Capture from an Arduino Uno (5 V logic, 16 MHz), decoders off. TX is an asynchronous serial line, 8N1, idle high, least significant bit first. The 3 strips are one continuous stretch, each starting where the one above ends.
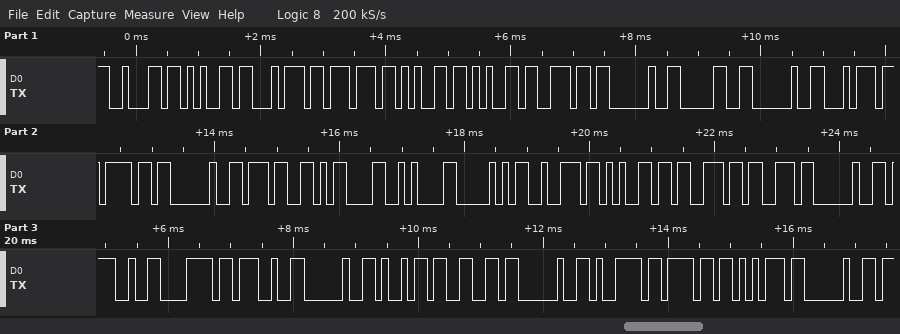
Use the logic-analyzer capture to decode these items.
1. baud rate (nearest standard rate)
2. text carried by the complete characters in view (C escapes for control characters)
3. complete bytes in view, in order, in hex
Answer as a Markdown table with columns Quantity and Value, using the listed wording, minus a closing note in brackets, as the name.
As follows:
| Quantity | Value |
|---|---|
| baud rate | 9600 baud |
| text carried by the complete characters in view | "between 0 to 7\r\nPress 'x' if you " |
| complete bytes in view, in order, in hex | 62 65 74 77 65 65 6E 20 30 20 74 6F 20 37 0D 0A 50 72 65 73 73 20 27 78 27 20 69 66 20 79 6F 75 20 |
